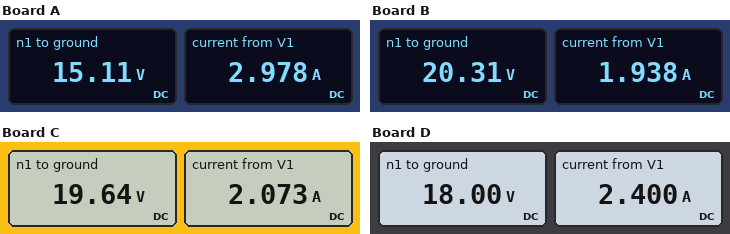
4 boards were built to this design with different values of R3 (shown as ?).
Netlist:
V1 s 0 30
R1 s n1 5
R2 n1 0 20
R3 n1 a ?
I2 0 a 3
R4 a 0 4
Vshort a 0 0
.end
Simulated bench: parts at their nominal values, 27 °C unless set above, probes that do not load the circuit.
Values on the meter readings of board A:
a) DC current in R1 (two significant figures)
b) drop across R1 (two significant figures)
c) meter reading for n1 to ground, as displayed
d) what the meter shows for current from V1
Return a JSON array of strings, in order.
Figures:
["3.0 A", "15 V", "15.11 V", "2.978 A"]
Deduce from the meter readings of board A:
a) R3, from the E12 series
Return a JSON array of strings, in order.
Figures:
["6.8 Ω"]
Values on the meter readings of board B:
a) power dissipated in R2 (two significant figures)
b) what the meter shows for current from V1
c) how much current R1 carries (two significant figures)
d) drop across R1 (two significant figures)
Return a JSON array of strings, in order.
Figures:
["21 W", "1.938 A", "1.9 A", "9.7 V"]
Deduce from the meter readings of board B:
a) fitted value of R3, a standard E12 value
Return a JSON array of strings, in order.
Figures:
["22 Ω"]
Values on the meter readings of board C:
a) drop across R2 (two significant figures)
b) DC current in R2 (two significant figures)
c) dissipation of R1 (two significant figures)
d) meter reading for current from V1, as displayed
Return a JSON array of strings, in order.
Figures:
["20 V", "980 mA", "21 W", "2.073 A"]
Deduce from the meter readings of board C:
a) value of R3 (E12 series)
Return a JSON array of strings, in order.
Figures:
["18 Ω"]
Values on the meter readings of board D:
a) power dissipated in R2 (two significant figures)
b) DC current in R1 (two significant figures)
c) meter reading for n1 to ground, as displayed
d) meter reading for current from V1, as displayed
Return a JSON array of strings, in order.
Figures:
["16 W", "2.4 A", "18.00 V", "2.400 A"]
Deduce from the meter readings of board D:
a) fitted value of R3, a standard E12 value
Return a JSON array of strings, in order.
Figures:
["12 Ω"]
